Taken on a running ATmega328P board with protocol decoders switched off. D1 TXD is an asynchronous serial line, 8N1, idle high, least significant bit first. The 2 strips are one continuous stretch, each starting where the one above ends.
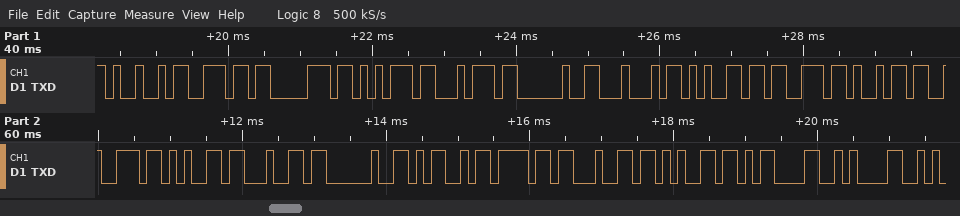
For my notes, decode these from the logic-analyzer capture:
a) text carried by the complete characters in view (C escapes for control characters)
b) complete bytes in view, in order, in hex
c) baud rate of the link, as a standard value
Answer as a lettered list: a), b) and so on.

a) "Input Desired Mode\r\n"
b) 0x49 0x6E 0x70 0x75 0x74 0x20 0x44 0x65 0x73 0x69 0x72 0x65 0x64 0x20 0x4D 0x6F 0x64 0x65 0x0D 0x0A
c) 9600 baud
